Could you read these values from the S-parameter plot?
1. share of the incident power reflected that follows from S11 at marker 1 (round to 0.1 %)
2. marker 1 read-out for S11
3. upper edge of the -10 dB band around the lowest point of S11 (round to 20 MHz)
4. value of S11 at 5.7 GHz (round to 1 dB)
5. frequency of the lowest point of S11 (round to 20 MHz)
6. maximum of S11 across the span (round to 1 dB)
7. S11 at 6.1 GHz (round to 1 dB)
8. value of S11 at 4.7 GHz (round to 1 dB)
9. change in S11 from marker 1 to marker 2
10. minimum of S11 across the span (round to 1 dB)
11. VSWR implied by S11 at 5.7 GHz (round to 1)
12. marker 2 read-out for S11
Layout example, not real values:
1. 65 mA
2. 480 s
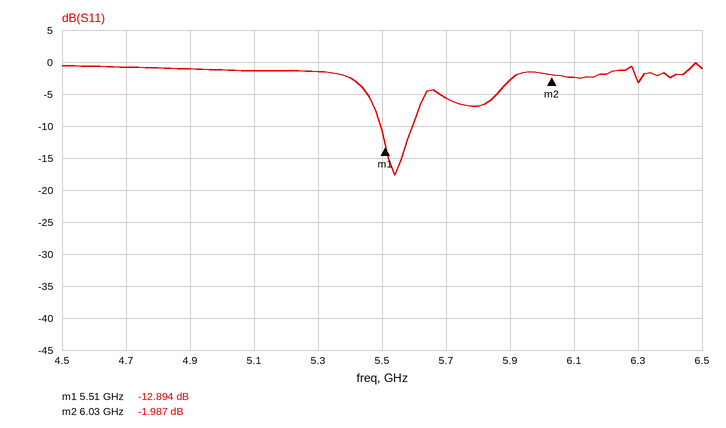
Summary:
1. 5.1 %
2. -12.894 dB
3. 5.60 GHz
4. -6 dB
5. 5.54 GHz
6. 0 dB
7. -2 dB
8. -1 dB
9. 10.907 dB
10. -18 dB
11. 3
12. -1.987 dB
